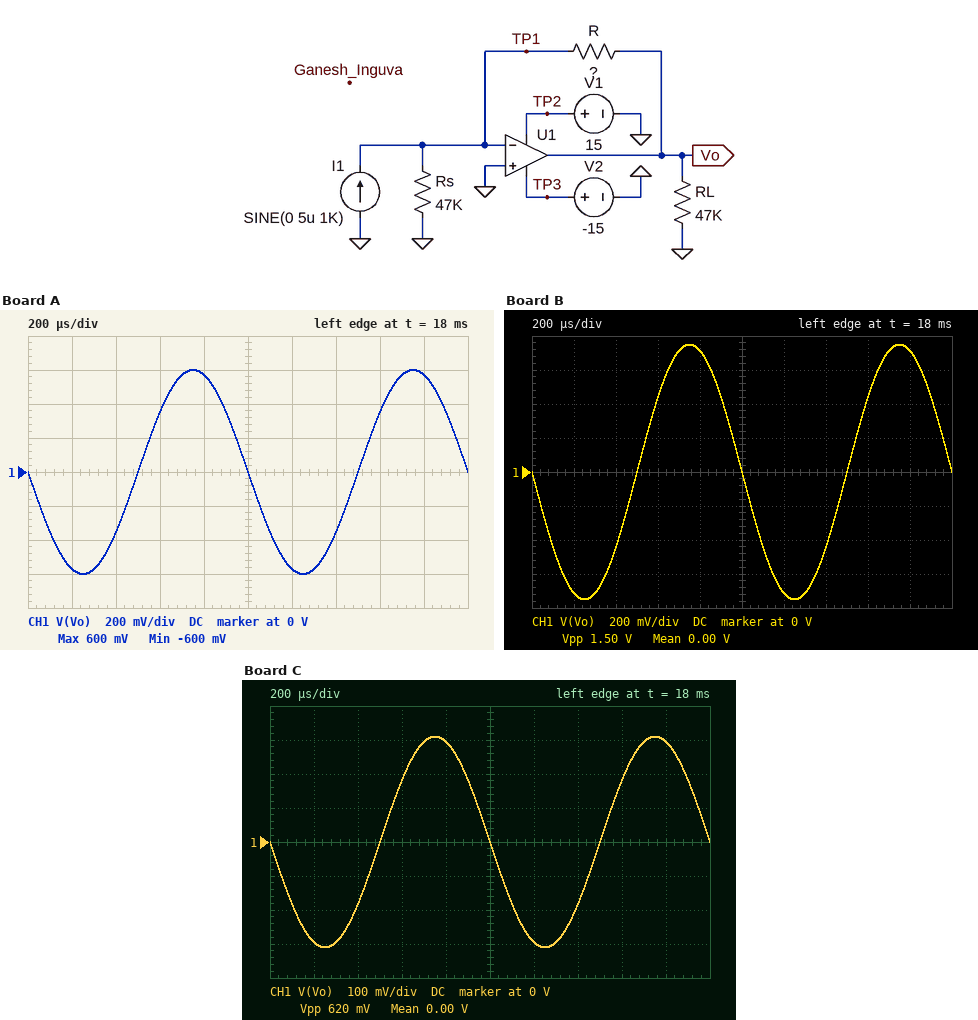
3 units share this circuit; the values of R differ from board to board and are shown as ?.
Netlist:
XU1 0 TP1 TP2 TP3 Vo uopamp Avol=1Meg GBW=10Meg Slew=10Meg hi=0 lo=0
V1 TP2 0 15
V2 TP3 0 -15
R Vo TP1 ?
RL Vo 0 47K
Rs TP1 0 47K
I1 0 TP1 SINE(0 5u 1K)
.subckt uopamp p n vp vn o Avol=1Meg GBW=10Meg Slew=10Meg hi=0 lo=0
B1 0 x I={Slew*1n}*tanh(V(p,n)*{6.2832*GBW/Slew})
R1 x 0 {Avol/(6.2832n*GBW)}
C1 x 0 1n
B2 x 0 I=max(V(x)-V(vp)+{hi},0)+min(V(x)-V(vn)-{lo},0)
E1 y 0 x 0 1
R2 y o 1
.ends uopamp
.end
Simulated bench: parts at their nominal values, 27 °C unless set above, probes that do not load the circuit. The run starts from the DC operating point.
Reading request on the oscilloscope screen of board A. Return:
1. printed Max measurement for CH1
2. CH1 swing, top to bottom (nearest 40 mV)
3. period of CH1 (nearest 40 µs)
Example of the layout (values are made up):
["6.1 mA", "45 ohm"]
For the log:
["600 mV", "1.20 V", "1.00 ms"]
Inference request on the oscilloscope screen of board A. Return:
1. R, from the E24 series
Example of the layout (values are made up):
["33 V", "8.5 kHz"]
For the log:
["120 kΩ"]
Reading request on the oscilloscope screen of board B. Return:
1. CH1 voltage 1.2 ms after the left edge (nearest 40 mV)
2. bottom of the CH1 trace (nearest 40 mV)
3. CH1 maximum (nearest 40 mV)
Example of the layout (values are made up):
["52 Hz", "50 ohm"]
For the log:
["-720 mV", "-760 mV", "760 mV"]
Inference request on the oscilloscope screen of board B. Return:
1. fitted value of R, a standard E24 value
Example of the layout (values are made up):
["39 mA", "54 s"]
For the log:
["150 kΩ"]
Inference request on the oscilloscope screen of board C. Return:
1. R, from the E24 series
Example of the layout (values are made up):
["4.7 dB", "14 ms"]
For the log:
["62 kΩ"]
